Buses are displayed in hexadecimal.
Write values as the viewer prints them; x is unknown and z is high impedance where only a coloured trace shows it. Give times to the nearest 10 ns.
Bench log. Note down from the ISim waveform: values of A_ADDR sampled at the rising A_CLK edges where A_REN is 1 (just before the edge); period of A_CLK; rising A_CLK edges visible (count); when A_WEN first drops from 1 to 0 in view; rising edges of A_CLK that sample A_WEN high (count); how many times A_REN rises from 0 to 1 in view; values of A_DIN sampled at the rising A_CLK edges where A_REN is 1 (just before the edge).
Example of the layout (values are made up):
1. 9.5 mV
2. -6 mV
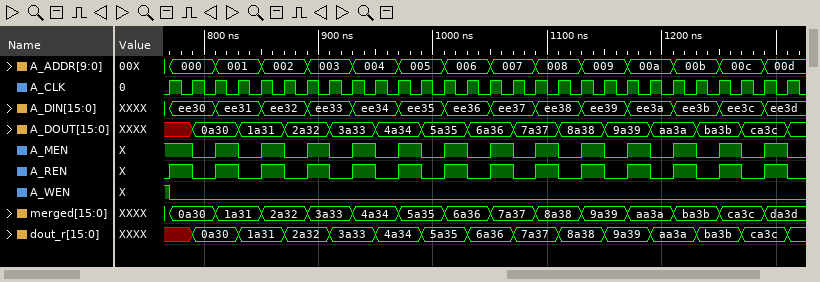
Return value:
1. 000, 001, 002, 003, 004, 005, 006, 007, 008, 009, 00a, 00b, 00c, 00d
2. 20 ns
3. 28
4. 770 ns
5. 1
6. 14
7. ee30, ee31, ee32, ee33, ee34, ee35, ee36, ee37, ee38, ee39, ee3a, ee3b, ee3c, ee3d
